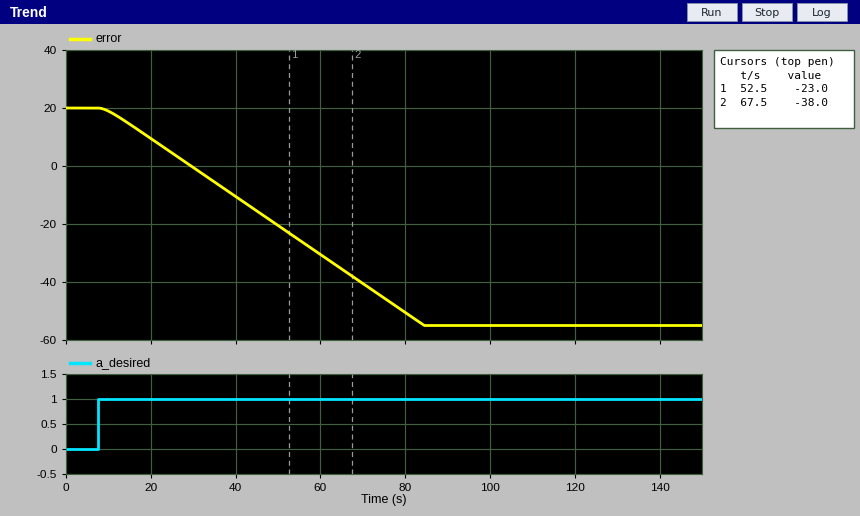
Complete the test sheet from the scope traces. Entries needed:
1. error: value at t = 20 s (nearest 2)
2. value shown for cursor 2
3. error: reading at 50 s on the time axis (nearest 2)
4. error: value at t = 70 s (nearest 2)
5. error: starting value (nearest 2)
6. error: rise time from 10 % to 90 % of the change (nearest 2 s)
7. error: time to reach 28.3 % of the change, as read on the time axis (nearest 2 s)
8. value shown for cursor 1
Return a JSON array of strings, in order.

["10", "-38.0", "-20", "-40", "20", "60 s", "30 s", "-23.0"]
